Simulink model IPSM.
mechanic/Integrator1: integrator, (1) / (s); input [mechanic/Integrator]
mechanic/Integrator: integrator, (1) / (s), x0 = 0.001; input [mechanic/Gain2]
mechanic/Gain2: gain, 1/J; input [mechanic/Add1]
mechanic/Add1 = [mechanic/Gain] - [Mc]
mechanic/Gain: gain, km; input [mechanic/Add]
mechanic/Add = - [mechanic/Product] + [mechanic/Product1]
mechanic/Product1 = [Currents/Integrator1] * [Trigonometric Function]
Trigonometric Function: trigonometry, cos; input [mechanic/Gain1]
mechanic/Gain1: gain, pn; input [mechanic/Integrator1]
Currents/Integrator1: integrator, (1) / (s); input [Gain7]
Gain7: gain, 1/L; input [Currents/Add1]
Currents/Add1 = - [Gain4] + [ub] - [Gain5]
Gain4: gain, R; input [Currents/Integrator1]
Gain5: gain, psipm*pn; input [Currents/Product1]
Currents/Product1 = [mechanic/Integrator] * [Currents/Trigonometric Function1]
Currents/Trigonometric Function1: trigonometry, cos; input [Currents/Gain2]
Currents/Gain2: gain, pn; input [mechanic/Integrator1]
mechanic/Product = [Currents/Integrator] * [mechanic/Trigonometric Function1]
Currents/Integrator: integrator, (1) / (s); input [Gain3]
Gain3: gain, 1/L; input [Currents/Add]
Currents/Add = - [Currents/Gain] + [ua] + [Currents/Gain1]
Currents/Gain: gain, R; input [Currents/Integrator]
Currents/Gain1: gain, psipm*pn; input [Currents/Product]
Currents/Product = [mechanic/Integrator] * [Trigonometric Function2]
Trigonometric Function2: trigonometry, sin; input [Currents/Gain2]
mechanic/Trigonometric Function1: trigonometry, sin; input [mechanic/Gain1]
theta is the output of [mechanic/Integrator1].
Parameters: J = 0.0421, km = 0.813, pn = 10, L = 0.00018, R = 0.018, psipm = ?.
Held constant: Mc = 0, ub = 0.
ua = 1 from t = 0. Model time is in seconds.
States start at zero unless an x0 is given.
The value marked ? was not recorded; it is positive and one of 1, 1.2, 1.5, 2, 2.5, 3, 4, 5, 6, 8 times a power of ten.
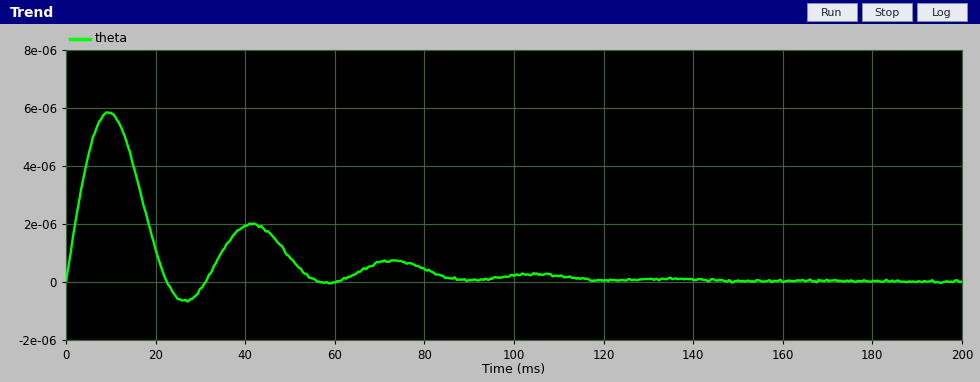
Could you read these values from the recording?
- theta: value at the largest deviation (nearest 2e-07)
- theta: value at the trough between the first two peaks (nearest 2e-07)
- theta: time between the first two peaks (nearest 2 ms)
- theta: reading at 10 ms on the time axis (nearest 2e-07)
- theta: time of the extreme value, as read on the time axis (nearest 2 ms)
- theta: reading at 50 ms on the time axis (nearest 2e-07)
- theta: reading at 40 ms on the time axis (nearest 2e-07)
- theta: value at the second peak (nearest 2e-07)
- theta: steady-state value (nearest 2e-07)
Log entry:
0.0000058
-0.0000006
32 ms
0.0000058
10 ms
0.0000008
0.0000020
0.0000020
0.0000000
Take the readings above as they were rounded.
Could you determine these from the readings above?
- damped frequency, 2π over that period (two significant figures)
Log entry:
0.20 rad/ms
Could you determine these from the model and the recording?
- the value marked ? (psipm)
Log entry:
0.03
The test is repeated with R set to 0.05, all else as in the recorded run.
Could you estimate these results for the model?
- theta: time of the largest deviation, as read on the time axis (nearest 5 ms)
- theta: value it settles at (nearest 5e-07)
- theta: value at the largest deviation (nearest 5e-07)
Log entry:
15 ms
0.0000000
0.0000075
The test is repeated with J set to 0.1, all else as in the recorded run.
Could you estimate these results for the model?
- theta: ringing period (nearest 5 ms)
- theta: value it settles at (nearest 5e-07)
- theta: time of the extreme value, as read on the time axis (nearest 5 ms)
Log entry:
50 ms
0.0000000
15 ms
